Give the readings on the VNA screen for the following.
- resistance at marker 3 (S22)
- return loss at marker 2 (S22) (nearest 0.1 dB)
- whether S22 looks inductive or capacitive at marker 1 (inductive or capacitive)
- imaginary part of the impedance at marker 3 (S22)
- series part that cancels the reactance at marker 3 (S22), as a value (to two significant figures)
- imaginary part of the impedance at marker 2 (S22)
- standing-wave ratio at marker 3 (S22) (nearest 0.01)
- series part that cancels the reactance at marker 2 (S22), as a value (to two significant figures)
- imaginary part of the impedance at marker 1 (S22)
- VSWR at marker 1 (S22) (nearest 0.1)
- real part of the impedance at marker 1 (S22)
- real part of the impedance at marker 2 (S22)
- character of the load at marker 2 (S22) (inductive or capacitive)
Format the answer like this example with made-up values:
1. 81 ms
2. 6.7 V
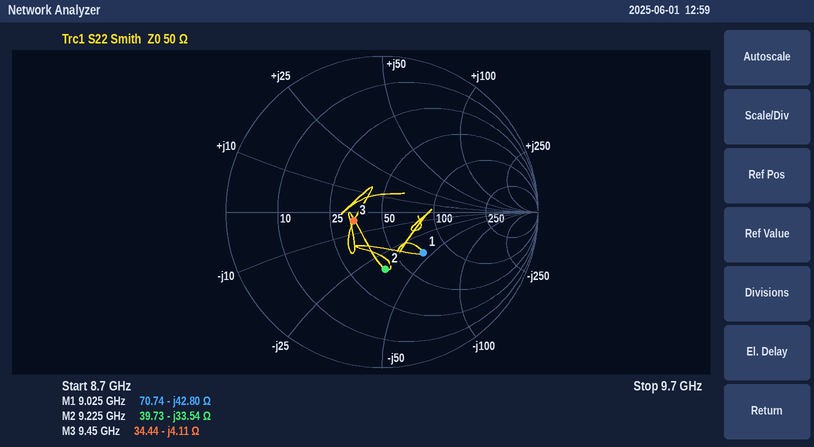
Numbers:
1. 34.44 Ω
2. 8.7 dB
3. capacitive
4. -4.11 Ω
5. 69 pH
6. -33.54 Ω
7. 1.47
8. 580 pH
9. -42.80 Ω
10. 2.2
11. 70.74 Ω
12. 39.73 Ω
13. capacitive
